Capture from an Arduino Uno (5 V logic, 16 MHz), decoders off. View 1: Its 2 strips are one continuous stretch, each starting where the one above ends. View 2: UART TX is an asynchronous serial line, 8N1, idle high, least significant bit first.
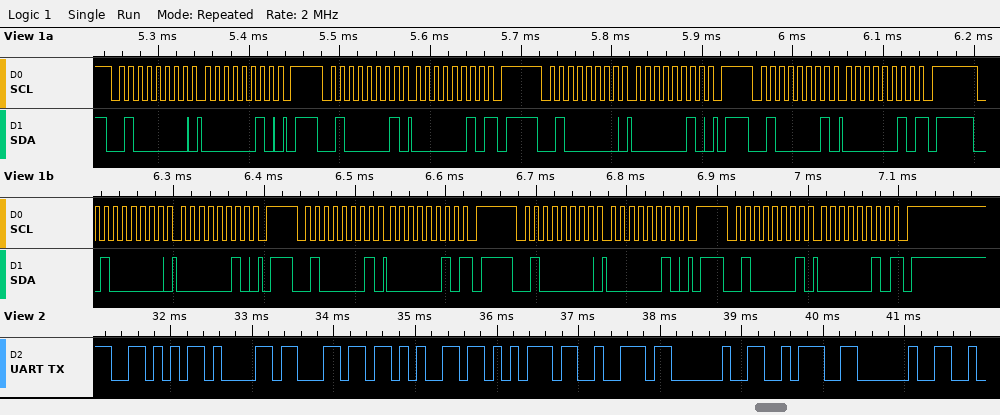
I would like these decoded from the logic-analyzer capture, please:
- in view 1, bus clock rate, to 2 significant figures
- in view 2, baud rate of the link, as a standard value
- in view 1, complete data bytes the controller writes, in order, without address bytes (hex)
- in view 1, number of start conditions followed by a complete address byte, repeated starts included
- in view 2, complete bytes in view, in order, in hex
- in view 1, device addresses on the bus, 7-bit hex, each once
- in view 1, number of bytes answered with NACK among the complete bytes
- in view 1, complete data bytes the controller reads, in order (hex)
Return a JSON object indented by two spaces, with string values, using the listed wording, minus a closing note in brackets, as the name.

{
  "in view 1, bus clock rate, to 2 significant figures": "100 kHz",
  "in view 2, baud rate of the link, as a standard value": "9600 baud",
  "in view 1, complete data bytes the controller writes, in order, without address bytes": "02 02 02 02",
  "in view 1, number of start conditions followed by a complete address byte, repeated starts included": "8",
  "in view 2, complete bytes in view, in order, in hex": "56 61 6C 65 75 72 20 3A 20",
  "in view 1, device addresses on the bus, 7-bit hex, each once": "0x20",
  "in view 1, number of bytes answered with NACK among the complete bytes": "4",
  "in view 1, complete data bytes the controller reads, in order": "02 02 02 02"
}
